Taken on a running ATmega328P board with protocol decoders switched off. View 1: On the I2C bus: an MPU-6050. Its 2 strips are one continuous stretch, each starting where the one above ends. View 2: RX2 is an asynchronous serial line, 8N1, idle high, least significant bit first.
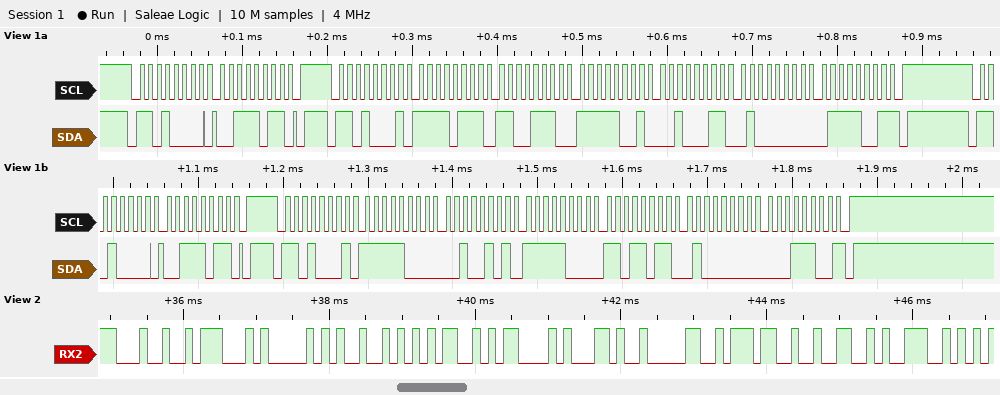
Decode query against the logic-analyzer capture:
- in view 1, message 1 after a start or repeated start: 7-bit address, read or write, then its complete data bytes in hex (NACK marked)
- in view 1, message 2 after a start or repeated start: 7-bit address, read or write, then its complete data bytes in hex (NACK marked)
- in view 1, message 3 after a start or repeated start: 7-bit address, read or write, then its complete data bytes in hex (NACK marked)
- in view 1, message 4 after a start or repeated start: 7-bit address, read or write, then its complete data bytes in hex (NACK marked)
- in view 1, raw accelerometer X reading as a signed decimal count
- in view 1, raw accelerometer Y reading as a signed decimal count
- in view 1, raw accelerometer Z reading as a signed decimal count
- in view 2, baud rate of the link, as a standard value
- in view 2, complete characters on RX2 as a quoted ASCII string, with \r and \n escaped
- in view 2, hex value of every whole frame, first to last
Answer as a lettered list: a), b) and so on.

a) 0x68 write: 3B
b) 0x68 read: F7 CE F9 23 40 79 NACK
c) 0x68 write: 3B
d) 0x68 read: F8 25 F8 DB 40 1C NACK
e) -2098
f) -1757
g) 16505
h) 9600 baud
i) "$GPRMC,0729"
j) 24 47 50 52 4D 43 2C 30 37 32 39
